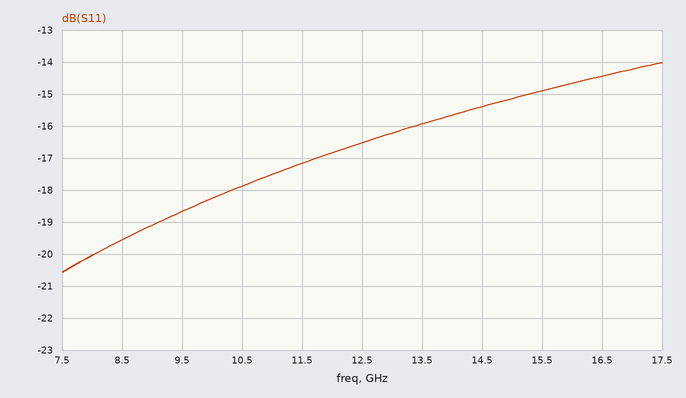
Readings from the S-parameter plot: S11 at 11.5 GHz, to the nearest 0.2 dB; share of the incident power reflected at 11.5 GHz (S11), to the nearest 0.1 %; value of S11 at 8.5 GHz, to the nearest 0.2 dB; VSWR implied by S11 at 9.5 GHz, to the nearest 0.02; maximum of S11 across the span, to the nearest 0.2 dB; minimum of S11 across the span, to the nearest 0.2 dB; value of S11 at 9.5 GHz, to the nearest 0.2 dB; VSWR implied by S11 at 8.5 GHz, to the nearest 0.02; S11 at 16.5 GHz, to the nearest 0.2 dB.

-17.2 dB
1.9 %
-19.6 dB
1.26
-14.0 dB
-20.6 dB
-18.6 dB
1.24
-14.4 dB
